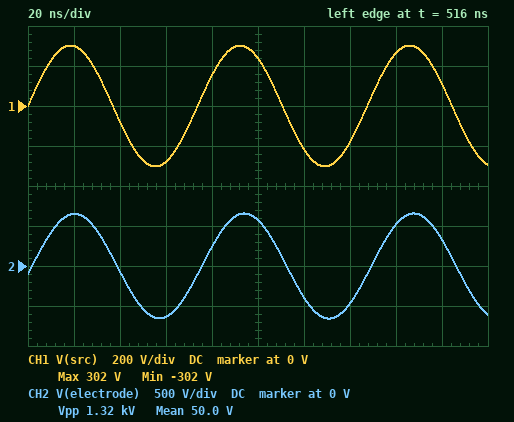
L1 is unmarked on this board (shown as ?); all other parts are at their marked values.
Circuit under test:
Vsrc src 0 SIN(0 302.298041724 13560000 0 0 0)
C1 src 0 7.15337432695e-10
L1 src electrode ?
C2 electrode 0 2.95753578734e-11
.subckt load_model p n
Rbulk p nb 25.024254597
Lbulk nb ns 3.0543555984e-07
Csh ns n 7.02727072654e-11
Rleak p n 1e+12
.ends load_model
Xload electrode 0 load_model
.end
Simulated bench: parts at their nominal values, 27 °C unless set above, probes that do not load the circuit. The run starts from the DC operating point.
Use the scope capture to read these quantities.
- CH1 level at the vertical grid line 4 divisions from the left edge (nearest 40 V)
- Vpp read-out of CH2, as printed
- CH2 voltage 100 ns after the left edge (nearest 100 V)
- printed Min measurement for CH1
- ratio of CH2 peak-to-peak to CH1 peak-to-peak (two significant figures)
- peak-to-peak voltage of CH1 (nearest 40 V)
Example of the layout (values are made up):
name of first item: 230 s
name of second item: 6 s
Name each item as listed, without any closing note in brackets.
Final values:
CH1 level at the vertical grid line 4 divisions from the left edge: 160 V
Vpp read-out of CH2, as printed: 1.32 kV
CH2 voltage 100 ns after the left edge: 600 V
printed Min measurement for CH1: -302 V
ratio of CH2 peak-to-peak to CH1 peak-to-peak: 2.2
peak-to-peak voltage of CH1: 600 V
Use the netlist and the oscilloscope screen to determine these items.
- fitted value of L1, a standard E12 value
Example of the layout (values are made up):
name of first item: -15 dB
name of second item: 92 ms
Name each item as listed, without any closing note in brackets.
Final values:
fitted value of L1, a standard E12 value: 680 nH
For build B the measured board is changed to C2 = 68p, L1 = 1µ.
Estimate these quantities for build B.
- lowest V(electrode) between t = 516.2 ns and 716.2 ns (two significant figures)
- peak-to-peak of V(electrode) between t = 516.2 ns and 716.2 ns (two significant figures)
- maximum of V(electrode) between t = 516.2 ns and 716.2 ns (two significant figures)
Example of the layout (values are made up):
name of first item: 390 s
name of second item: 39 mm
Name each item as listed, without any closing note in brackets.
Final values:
lowest V(electrode) between t = 516.2 ns and 716.2 ns: -2.5 kV
peak-to-peak of V(electrode) between t = 516.2 ns and 716.2 ns: 5.0 kV
maximum of V(electrode) between t = 516.2 ns and 716.2 ns: 2.5 kV
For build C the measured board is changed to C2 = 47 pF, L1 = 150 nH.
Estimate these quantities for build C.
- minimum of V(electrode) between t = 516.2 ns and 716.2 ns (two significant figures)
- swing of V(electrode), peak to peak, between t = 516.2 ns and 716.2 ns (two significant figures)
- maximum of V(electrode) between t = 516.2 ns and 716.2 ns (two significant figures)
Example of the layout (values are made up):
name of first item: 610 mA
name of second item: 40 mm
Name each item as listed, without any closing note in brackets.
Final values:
minimum of V(electrode) between t = 516.2 ns and 716.2 ns: -350 V
swing of V(electrode), peak to peak, between t = 516.2 ns and 716.2 ns: 700 V
maximum of V(electrode) between t = 516.2 ns and 716.2 ns: 350 V
